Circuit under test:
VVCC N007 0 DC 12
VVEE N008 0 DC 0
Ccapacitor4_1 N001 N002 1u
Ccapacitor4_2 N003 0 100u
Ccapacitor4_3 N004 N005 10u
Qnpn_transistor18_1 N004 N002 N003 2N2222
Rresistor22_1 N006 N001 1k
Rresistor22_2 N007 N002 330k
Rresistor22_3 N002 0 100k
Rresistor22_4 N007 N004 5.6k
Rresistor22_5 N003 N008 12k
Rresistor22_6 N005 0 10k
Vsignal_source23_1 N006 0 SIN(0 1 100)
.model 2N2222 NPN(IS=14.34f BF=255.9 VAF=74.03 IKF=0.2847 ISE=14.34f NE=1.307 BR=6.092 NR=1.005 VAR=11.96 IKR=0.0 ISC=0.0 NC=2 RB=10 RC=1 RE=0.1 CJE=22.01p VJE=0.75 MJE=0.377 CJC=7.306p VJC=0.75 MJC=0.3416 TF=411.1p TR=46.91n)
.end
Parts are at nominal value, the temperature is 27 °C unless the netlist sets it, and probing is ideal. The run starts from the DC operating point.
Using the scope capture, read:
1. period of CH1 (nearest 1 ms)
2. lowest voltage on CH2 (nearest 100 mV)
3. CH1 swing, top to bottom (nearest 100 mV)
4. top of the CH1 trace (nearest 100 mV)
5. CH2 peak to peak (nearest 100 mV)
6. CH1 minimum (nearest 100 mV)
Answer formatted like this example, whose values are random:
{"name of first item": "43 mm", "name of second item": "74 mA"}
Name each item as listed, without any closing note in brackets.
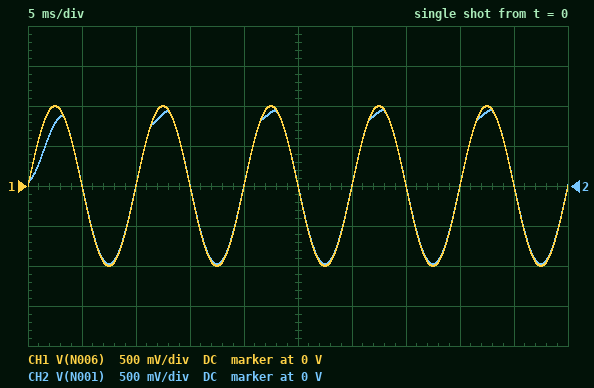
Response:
{"period of CH1": "10 ms", "lowest voltage on CH2": "-1.0 V", "CH1 swing, top to bottom": "2.0 V", "top of the CH1 trace": "1.0 V", "CH2 peak to peak": "1.9 V", "CH1 minimum": "-1.0 V"}
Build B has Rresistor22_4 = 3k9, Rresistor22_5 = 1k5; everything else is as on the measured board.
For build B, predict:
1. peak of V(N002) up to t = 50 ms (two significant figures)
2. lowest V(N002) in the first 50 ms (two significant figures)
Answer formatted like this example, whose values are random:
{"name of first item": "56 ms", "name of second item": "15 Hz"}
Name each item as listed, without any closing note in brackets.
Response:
{"peak of V(N002) up to t = 50 ms": "2.4 V", "lowest V(N002) in the first 50 ms": "410 mV"}
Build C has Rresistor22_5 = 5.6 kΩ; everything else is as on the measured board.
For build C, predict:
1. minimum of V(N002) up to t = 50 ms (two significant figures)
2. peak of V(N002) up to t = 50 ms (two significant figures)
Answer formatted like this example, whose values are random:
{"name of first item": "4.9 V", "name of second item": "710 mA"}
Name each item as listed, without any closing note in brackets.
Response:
{"minimum of V(N002) up to t = 50 ms": "890 mV", "peak of V(N002) up to t = 50 ms": "2.8 V"}
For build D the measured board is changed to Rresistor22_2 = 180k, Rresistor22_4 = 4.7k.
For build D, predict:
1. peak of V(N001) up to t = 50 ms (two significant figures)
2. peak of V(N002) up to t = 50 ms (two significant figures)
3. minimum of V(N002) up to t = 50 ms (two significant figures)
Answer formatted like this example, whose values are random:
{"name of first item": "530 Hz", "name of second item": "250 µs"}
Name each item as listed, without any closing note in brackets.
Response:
{"peak of V(N001) up to t = 50 ms": "940 mV", "peak of V(N002) up to t = 50 ms": "4.3 V", "minimum of V(N002) up to t = 50 ms": "2.5 V"}
